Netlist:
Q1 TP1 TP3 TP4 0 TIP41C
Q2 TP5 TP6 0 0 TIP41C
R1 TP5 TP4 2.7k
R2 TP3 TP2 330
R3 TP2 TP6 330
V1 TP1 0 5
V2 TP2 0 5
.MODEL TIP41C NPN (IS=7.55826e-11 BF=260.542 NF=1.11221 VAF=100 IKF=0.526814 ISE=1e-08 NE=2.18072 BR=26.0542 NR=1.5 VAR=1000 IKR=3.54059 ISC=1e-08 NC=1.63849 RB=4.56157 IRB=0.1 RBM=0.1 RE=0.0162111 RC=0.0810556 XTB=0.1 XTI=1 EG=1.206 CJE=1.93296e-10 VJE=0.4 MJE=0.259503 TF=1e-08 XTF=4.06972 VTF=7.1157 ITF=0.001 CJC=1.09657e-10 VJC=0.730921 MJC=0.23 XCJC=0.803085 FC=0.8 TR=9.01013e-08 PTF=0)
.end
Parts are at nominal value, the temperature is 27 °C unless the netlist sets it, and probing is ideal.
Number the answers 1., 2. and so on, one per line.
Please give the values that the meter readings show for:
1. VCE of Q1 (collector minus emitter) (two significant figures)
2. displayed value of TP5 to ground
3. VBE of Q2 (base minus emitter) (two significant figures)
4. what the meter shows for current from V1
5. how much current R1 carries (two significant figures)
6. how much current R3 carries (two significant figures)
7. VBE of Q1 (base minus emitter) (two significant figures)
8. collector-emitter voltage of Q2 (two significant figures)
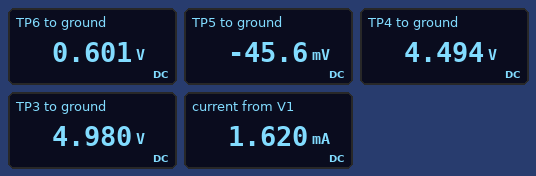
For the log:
1. 510 mV
2. -45.6 mV
3. 600 mV
4. 1.620 mA
5. 1.7 mA
6. 13 mA
7. 490 mV
8. -46 mV
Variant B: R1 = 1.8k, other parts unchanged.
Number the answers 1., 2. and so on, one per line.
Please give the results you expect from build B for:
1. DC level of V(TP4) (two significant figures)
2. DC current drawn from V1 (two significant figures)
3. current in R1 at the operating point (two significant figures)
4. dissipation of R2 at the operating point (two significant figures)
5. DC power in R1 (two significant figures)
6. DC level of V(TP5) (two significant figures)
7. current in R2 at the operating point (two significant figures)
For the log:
1. 4.5 V
2. 2.4 mA
3. 2.5 mA
4. 2.0 µW
5. 11 mW
6. -44 mV
7. 77 µA
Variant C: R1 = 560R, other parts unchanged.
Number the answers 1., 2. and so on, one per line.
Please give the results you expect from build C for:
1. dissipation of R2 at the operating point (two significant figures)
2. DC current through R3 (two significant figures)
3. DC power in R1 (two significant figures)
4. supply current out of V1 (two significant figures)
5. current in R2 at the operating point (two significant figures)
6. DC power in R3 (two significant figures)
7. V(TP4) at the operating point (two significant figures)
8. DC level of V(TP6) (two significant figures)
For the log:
1. 7.8 µW
2. 13 mA
3. 35 mW
4. 7.8 mA
5. 150 µA
6. 58 mW
7. 4.4 V
8. 610 mV
